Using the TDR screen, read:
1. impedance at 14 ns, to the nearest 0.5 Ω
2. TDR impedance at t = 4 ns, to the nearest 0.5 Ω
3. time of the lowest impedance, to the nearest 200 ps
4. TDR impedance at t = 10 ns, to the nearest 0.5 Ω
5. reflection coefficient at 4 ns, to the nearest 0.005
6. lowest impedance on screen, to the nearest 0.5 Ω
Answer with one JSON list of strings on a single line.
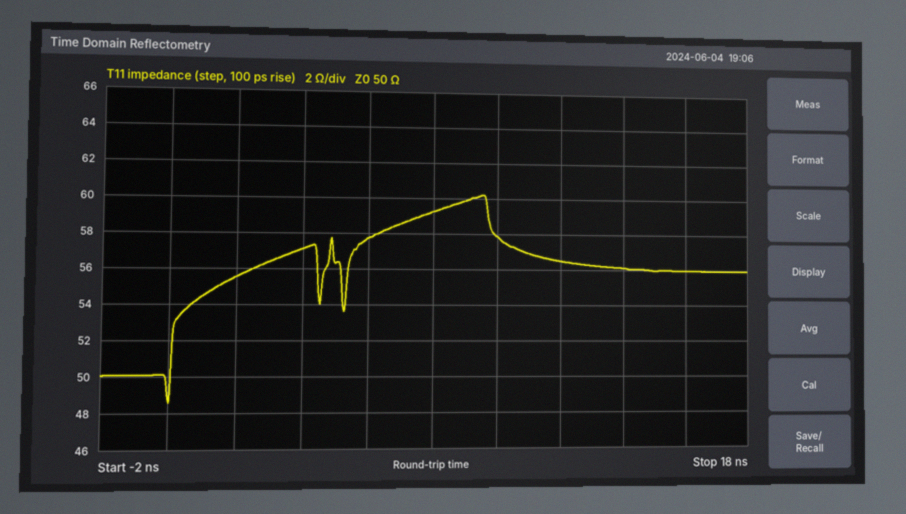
["56.0 Ω", "57.0 Ω", "0.0 ns", "58.0 Ω", "+0.065", "48.5 Ω"]
